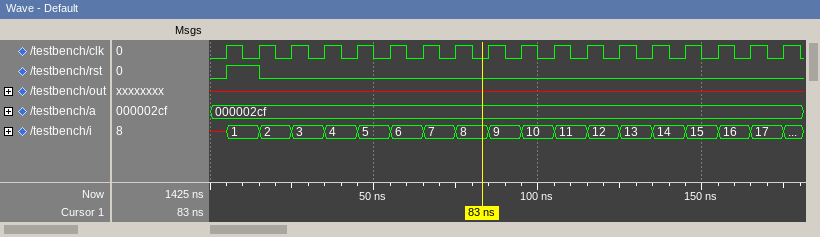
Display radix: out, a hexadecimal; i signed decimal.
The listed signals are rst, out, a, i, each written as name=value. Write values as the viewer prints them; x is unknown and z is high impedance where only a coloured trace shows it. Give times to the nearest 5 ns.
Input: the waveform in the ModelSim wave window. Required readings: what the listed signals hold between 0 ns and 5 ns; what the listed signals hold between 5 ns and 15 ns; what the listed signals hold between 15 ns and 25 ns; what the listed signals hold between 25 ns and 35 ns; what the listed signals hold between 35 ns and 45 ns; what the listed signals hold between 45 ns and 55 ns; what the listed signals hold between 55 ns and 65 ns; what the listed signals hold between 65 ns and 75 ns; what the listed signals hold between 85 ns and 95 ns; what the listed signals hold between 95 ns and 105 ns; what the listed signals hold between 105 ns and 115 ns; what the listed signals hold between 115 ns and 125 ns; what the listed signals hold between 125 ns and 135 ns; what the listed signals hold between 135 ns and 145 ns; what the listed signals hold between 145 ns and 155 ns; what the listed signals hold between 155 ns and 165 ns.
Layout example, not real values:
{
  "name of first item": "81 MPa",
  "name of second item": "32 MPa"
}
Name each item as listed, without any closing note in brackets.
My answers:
{
  "what the listed signals hold between 0 ns and 5 ns": "rst=0, out=x, a=000002cf, i=x",
  "what the listed signals hold between 5 ns and 15 ns": "rst=1, out=x, a=000002cf, i=1",
  "what the listed signals hold between 15 ns and 25 ns": "rst=0, out=x, a=000002cf, i=2",
  "what the listed signals hold between 25 ns and 35 ns": "rst=0, out=x, a=000002cf, i=3",
  "what the listed signals hold between 35 ns and 45 ns": "rst=0, out=x, a=000002cf, i=4",
  "what the listed signals hold between 45 ns and 55 ns": "rst=0, out=x, a=000002cf, i=5",
  "what the listed signals hold between 55 ns and 65 ns": "rst=0, out=x, a=000002cf, i=6",
  "what the listed signals hold between 65 ns and 75 ns": "rst=0, out=x, a=000002cf, i=7",
  "what the listed signals hold between 85 ns and 95 ns": "rst=0, out=x, a=000002cf, i=9",
  "what the listed signals hold between 95 ns and 105 ns": "rst=0, out=x, a=000002cf, i=10",
  "what the listed signals hold between 105 ns and 115 ns": "rst=0, out=x, a=000002cf, i=11",
  "what the listed signals hold between 115 ns and 125 ns": "rst=0, out=x, a=000002cf, i=12",
  "what the listed signals hold between 125 ns and 135 ns": "rst=0, out=x, a=000002cf, i=13",
  "what the listed signals hold between 135 ns and 145 ns": "rst=0, out=x, a=000002cf, i=14",
  "what the listed signals hold between 145 ns and 155 ns": "rst=0, out=x, a=000002cf, i=15",
  "what the listed signals hold between 155 ns and 165 ns": "rst=0, out=x, a=000002cf, i=16"
}
